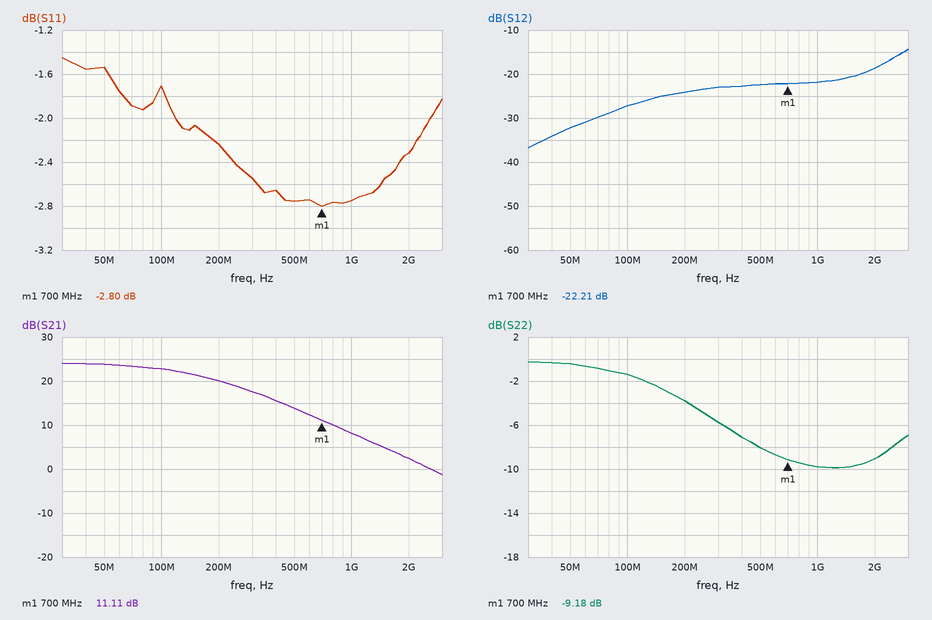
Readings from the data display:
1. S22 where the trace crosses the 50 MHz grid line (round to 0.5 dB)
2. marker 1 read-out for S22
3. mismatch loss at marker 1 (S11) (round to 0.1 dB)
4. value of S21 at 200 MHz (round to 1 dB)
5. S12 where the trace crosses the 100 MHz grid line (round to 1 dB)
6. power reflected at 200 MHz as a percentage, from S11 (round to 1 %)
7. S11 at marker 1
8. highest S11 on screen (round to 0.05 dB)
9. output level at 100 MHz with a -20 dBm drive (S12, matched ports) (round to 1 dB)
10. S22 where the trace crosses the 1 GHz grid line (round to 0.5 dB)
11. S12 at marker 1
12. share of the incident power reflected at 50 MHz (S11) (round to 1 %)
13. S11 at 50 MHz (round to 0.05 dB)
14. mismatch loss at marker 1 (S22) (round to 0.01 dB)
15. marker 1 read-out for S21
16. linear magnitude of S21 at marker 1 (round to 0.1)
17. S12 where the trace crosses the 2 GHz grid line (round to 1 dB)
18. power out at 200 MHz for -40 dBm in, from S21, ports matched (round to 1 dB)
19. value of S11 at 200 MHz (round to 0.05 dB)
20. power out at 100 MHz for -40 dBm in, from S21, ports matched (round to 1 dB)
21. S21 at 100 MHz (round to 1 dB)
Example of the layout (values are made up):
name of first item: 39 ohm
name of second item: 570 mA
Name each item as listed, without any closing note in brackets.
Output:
S22 where the trace crosses the 50 MHz grid line: -0.5 dB
marker 1 read-out for S22: -9.18 dB
mismatch loss at marker 1 (S11): 3.2 dB
value of S21 at 200 MHz: 20 dB
S12 where the trace crosses the 100 MHz grid line: -27 dB
power reflected at 200 MHz as a percentage, from S11: 60 %
S11 at marker 1: -2.80 dB
highest S11 on screen: -1.45 dB
output level at 100 MHz with a -20 dBm drive (S12, matched ports): -47 dBm
S22 where the trace crosses the 1 GHz grid line: -10.0 dB
S12 at marker 1: -22.21 dB
share of the incident power reflected at 50 MHz (S11): 70 %
S11 at 50 MHz: -1.55 dB
mismatch loss at marker 1 (S22): 0.56 dB
marker 1 read-out for S21: 11.11 dB
linear magnitude of S21 at marker 1: 3.6
S12 where the trace crosses the 2 GHz grid line: -19 dB
power out at 200 MHz for -40 dBm in, from S21, ports matched: -20 dBm
value of S11 at 200 MHz: -2.25 dB
power out at 100 MHz for -40 dBm in, from S21, ports matched: -17 dBm
S21 at 100 MHz: 23 dB
